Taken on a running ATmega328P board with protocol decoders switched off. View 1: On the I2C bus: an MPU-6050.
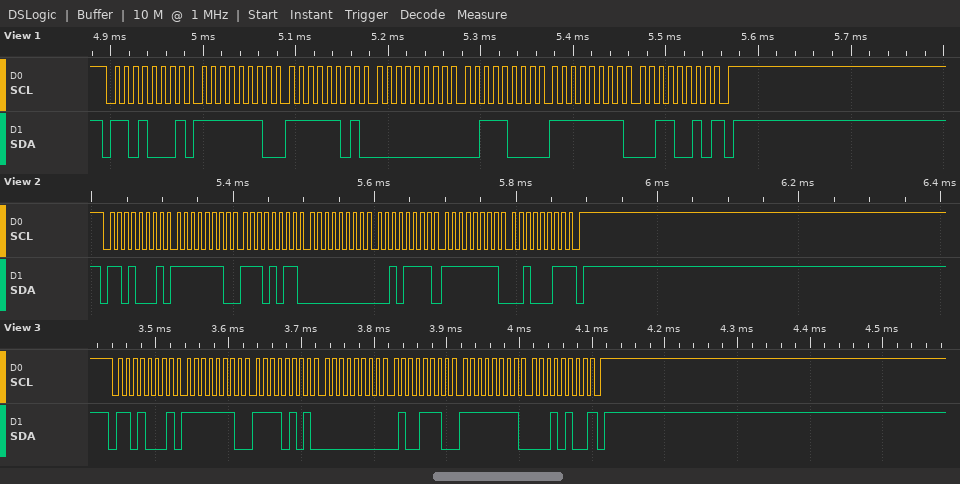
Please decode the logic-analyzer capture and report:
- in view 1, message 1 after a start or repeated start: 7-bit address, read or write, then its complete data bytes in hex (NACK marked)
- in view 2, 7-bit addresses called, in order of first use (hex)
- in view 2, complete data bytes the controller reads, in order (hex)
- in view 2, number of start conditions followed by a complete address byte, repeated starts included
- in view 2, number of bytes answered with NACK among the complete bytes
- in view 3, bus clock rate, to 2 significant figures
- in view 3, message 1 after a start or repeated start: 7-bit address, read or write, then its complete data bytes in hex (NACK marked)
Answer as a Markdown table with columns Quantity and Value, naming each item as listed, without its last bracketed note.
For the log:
| Quantity | Value |
|---|---|
| in view 1, message 1 after a start or repeated start: 7-bit address, read or write, then its complete data bytes in hex | 0x68 read: FE FD 00 38 FF 32 NACK |
| in view 2, 7-bit addresses called, in order of first use | 0x68 |
| in view 2, complete data bytes the controller reads, in order | FE EB 00 2F FF 23 |
| in view 2, number of start conditions followed by a complete address byte, repeated starts included | 1 |
| in view 2, number of bytes answered with NACK among the complete bytes | 1 |
| in view 3, bus clock rate, to 2 significant figures | 100 kHz |
| in view 3, message 1 after a start or repeated start: 7-bit address, read or write, then its complete data bytes in hex | 0x68 read: FE F5 00 4E FF 14 NACK |
